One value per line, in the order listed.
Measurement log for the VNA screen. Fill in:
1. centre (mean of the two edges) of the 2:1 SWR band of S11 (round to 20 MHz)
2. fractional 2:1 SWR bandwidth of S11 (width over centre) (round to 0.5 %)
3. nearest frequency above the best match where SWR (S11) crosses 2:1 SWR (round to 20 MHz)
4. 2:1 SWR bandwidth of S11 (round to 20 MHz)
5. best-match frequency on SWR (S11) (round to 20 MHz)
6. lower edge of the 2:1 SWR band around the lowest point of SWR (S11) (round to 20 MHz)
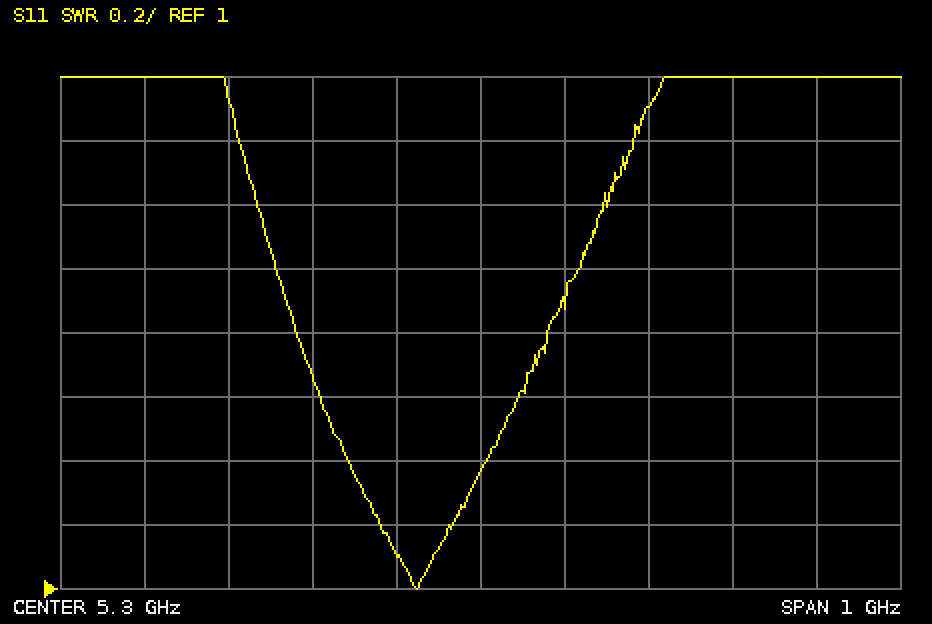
5.24 GHz
7.0 %
5.42 GHz
360 MHz
5.22 GHz
5.06 GHz
